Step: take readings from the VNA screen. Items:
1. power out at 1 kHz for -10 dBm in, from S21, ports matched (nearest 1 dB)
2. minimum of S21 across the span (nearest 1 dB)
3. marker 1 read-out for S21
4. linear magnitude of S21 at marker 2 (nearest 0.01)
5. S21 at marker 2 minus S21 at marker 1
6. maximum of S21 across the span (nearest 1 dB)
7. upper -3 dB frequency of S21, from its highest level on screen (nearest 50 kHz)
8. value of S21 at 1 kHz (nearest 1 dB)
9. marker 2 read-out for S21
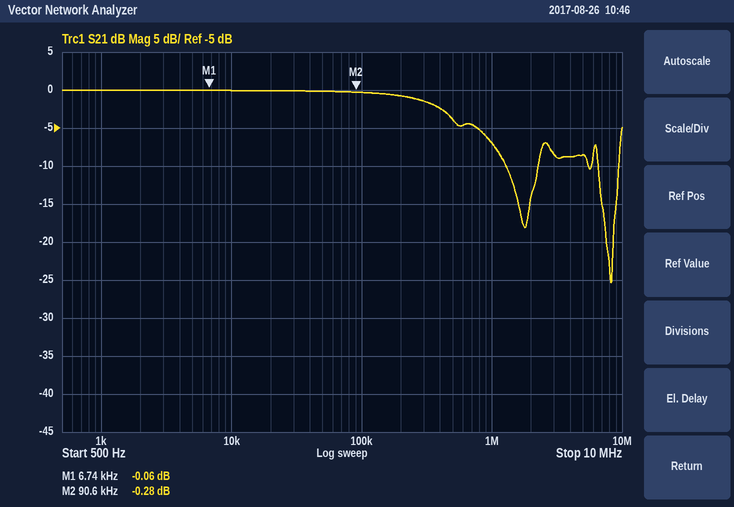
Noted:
-10 dBm
-25 dB
-0.06 dB
0.97
-0.22 dB
0 dB
450 kHz
0 dB
-0.28 dB
